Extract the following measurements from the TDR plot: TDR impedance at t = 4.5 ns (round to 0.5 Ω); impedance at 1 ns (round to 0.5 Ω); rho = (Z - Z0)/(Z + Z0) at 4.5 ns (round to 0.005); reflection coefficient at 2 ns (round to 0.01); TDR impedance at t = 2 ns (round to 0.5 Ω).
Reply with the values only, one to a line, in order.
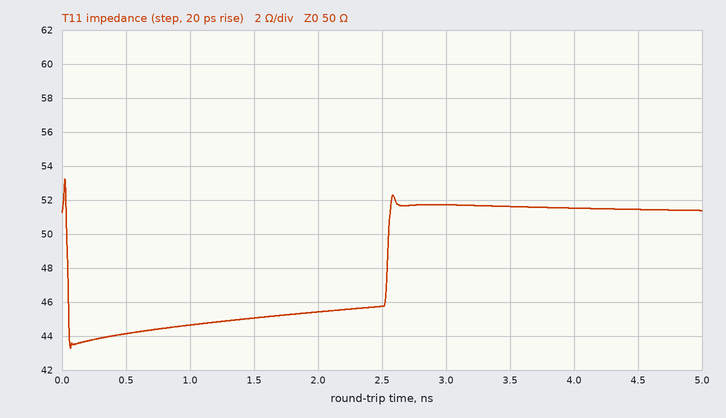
51.5 Ω
44.5 Ω
+0.015
-0.05
45.5 Ω
